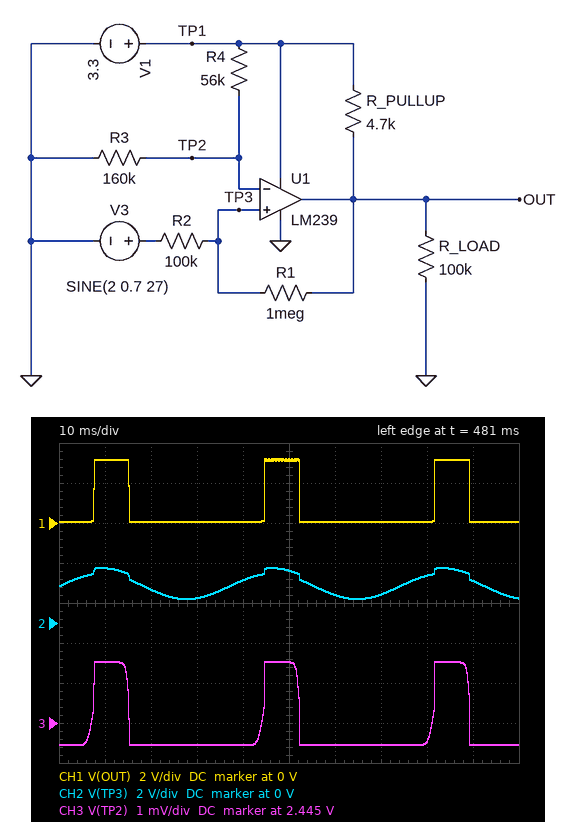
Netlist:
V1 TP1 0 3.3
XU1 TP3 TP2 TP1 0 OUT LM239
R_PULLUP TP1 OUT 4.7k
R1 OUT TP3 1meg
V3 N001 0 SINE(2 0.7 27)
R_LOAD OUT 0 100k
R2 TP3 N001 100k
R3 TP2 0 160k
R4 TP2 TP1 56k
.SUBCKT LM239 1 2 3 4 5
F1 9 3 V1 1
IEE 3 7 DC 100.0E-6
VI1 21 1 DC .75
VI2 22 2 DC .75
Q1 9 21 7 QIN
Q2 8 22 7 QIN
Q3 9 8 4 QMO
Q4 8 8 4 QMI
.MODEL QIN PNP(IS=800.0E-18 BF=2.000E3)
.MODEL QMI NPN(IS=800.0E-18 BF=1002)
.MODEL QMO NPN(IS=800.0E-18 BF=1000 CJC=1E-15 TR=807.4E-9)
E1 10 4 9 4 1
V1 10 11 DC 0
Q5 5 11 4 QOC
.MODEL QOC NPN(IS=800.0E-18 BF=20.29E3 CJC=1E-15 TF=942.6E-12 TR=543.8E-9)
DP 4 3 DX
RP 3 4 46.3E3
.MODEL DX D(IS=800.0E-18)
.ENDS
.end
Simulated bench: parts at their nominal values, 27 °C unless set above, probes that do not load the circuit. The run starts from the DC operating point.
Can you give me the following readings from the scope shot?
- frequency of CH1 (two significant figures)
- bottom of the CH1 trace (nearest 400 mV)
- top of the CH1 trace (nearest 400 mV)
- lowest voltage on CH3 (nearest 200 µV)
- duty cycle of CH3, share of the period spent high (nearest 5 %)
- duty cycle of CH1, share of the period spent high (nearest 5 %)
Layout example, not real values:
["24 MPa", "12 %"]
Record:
["27 Hz", "0 V", "3.2 V", "2.4444 V", "20 %", "20 %"]
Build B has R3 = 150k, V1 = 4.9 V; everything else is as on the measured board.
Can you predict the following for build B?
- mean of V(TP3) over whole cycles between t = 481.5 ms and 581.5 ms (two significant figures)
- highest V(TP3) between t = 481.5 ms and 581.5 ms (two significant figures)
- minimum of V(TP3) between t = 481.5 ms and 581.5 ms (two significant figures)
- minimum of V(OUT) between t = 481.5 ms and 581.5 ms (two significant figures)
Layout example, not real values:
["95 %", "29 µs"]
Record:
["1.8 V", "2.5 V", "1.2 V", "65 mV"]
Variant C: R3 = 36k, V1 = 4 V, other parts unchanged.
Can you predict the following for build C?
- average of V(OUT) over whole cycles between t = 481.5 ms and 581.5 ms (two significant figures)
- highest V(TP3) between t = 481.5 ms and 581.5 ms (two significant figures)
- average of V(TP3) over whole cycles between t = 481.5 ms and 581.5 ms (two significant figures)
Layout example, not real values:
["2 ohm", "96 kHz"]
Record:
["2.9 V", "2.8 V", "2.1 V"]
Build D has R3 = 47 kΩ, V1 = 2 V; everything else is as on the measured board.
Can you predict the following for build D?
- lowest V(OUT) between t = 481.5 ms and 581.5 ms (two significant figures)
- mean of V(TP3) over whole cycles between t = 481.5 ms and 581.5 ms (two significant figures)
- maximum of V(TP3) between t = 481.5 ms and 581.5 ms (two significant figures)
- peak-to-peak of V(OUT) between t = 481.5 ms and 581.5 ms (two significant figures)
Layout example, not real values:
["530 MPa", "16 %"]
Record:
["1.9 V", "2.0 V", "2.6 V", "5.7 mV"]
